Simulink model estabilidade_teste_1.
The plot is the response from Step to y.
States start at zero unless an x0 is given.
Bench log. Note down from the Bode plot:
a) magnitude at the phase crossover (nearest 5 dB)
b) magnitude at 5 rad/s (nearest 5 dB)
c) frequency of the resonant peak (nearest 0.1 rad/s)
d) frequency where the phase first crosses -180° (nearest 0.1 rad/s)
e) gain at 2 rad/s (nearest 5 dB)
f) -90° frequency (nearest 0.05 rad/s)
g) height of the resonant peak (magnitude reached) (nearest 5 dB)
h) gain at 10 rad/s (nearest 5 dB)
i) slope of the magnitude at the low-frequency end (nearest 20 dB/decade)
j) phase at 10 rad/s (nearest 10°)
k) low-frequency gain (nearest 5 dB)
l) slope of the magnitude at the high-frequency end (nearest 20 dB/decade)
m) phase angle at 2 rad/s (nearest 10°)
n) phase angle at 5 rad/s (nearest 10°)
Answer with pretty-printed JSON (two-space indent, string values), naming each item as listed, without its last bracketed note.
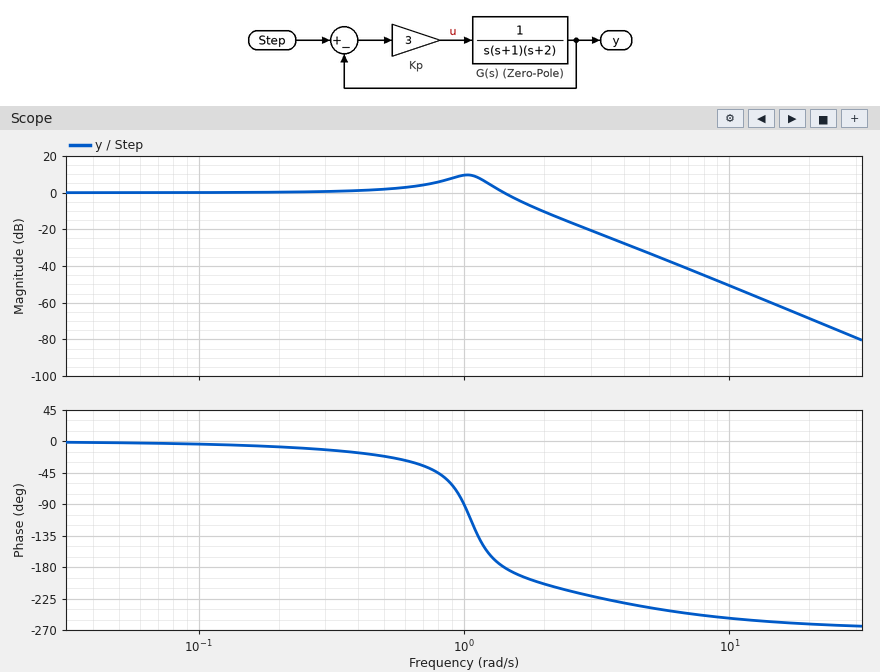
{
  "magnitude at the phase crossover": "0 dB",
  "magnitude at 5 rad/s": "-35 dB",
  "frequency of the resonant peak": "1.0 rad/s",
  "frequency where the phase first crosses -180°": "1.4 rad/s",
  "gain at 2 rad/s": "-10 dB",
  "-90° frequency": "1.00 rad/s",
  "height of the resonant peak (magnitude reached)": "10 dB",
  "gain at 10 rad/s": "-50 dB",
  "slope of the magnitude at the low-frequency end": "0 dB/decade",
  "phase at 10 rad/s": "-250°",
  "low-frequency gain": "0 dB",
  "slope of the magnitude at the high-frequency end": "-60 dB/decade",
  "phase angle at 2 rad/s": "-200°",
  "phase angle at 5 rad/s": "-240°"
}
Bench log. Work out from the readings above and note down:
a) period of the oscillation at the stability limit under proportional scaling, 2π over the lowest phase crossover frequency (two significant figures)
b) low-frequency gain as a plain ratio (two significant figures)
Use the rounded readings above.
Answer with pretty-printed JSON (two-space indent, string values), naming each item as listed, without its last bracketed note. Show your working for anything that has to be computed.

{
  "period of the oscillation at the stability limit under proportional scaling, 2π over the lowest phase crossover frequency": "2π / 1.4 = 4.5 s",
  "low-frequency gain as a plain ratio": "10^(0 / 20) = 1.0"
}
